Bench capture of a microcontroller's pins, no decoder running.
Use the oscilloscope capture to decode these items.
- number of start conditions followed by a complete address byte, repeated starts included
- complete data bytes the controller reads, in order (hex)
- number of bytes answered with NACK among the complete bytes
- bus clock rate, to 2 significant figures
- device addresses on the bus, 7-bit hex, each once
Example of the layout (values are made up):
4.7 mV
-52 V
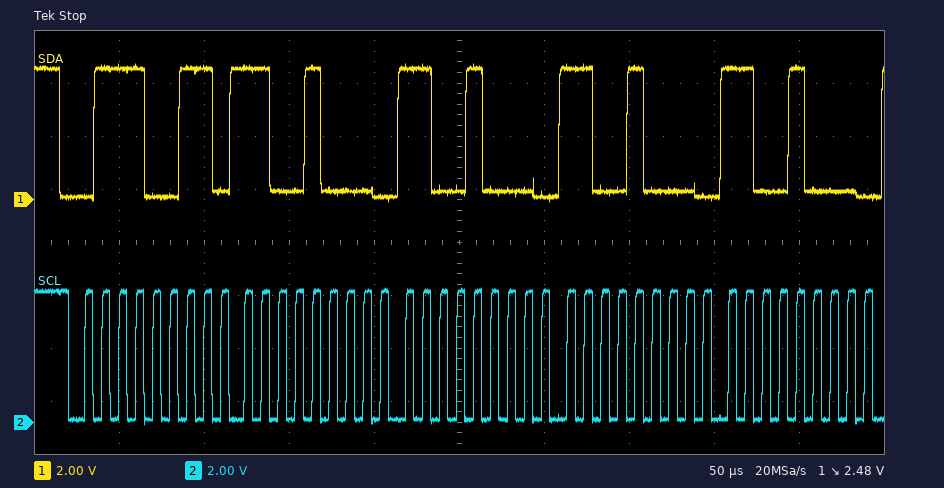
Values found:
1
C8 C8 C8 C8
0
100 kHz
0x39
